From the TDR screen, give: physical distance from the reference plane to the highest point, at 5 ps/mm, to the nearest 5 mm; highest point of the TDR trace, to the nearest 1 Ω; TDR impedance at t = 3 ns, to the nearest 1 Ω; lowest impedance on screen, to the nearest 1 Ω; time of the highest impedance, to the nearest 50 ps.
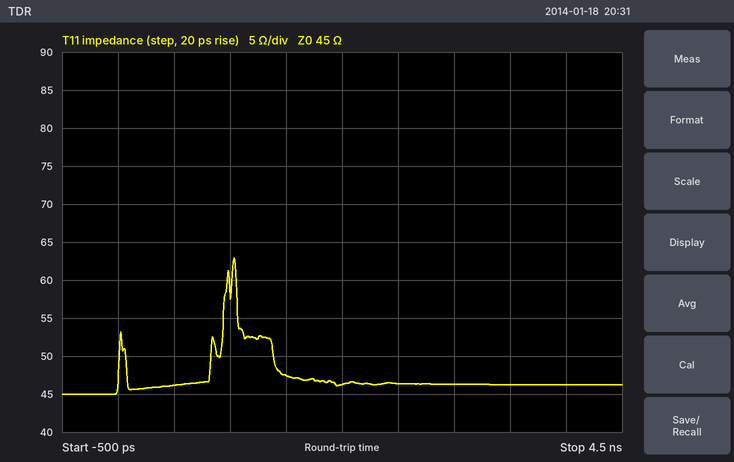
105 mm
63 Ω
46 Ω
45 Ω
1.05 ns
